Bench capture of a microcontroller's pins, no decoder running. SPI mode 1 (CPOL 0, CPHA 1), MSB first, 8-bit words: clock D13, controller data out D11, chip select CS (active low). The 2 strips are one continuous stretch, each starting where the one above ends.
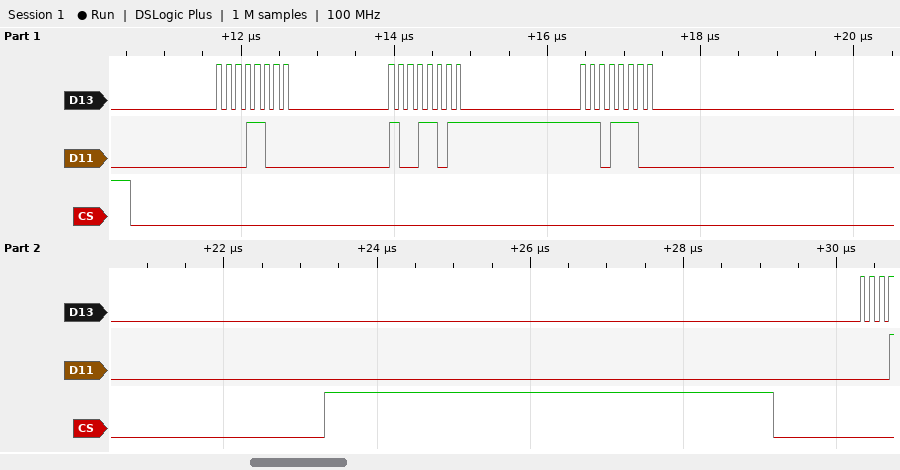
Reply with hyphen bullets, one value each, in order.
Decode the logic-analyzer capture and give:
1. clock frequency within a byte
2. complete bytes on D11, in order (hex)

- 8 MHz
- 18 9B DC
